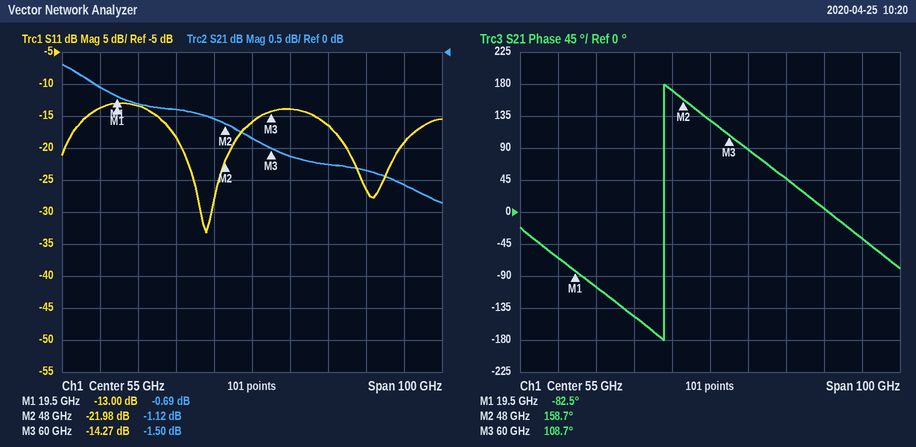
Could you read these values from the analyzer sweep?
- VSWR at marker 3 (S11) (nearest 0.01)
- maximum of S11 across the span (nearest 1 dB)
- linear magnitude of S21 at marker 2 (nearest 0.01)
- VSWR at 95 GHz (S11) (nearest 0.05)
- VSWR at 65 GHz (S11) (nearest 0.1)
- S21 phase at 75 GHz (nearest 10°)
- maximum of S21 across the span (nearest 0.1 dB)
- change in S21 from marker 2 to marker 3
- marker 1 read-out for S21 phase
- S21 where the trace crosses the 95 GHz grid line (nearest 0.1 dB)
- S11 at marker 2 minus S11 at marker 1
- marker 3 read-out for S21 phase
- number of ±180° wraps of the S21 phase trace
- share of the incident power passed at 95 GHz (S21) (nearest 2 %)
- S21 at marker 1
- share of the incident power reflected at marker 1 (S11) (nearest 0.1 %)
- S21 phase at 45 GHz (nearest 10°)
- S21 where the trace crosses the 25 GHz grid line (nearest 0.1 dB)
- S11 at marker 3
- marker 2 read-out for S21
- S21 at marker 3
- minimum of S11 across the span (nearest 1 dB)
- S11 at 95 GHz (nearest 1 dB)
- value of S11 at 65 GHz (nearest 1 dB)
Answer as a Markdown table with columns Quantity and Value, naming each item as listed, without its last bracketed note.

| Quantity | Value |
|---|---|
| VSWR at marker 3 (S11) | 1.48 |
| maximum of S11 across the span | -13 dB |
| linear magnitude of S21 at marker 2 | 0.88 |
| VSWR at 95 GHz (S11) | 1.25 |
| VSWR at 65 GHz (S11) | 1.5 |
| S21 phase at 75 GHz | 50° |
| maximum of S21 across the span | -0.2 dB |
| change in S21 from marker 2 to marker 3 | -0.38 dB |
| marker 1 read-out for S21 phase | -82.5° |
| S21 where the trace crosses the 95 GHz grid line | -2.1 dB |
| S11 at marker 2 minus S11 at marker 1 | -8.98 dB |
| marker 3 read-out for S21 phase | 108.7° |
| number of ±180° wraps of the S21 phase trace | 1 |
| share of the incident power passed at 95 GHz (S21) | 62 % |
| S21 at marker 1 | -0.69 dB |
| share of the incident power reflected at marker 1 (S11) | 5.0 % |
| S21 phase at 45 GHz | 170° |
| S21 where the trace crosses the 25 GHz grid line | -0.8 dB |
| S11 at marker 3 | -14.27 dB |
| marker 2 read-out for S21 | -1.12 dB |
| S21 at marker 3 | -1.50 dB |
| minimum of S11 across the span | -33 dB |
| S11 at 95 GHz | -19 dB |
| value of S11 at 65 GHz | -14 dB |
